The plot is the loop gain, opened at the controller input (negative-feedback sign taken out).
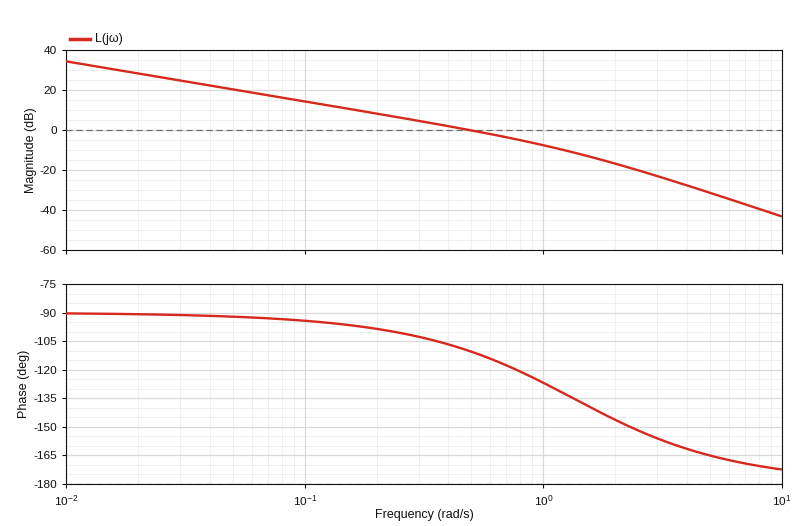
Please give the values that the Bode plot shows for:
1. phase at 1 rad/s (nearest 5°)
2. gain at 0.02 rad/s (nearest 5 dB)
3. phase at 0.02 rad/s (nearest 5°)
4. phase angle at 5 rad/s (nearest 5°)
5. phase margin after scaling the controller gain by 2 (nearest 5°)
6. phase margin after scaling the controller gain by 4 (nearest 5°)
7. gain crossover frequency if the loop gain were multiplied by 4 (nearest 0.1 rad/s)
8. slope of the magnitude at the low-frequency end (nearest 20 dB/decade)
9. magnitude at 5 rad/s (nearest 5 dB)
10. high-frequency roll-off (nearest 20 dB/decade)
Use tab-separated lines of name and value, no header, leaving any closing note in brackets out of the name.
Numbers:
phase at 1 rad/s	-125°
gain at 0.02 rad/s	30 dB
phase at 0.02 rad/s	-90°
phase angle at 5 rad/s	-165°
phase margin after scaling the controller gain by 2	55°
phase margin after scaling the controller gain by 4	45°
gain crossover frequency if the loop gain were multiplied by 4	1.4 rad/s
slope of the magnitude at the low-frequency end	-20 dB/decade
magnitude at 5 rad/s	-30 dB
high-frequency roll-off	-40 dB/decade
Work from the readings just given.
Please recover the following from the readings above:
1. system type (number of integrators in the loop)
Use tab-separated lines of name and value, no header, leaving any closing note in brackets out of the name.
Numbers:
system type	1
